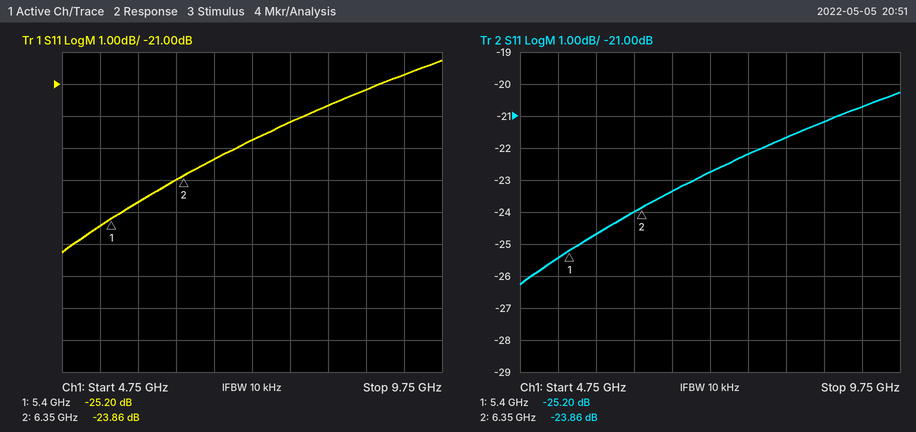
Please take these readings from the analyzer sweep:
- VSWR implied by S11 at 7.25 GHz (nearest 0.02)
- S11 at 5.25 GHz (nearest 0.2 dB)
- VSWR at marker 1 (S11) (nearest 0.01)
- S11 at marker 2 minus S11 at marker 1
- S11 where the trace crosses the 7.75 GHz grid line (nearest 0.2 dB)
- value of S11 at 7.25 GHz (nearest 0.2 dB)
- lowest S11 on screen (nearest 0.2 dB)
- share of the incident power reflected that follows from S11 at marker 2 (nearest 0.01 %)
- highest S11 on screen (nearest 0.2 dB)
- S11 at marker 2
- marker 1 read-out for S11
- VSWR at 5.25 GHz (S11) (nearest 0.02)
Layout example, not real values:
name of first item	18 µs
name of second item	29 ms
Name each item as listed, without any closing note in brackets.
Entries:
VSWR implied by S11 at 7.25 GHz	1.16
S11 at 5.25 GHz	-25.4 dB
VSWR at marker 1 (S11)	1.12
S11 at marker 2 minus S11 at marker 1	1.34 dB
S11 where the trace crosses the 7.75 GHz grid line	-22.2 dB
value of S11 at 7.25 GHz	-22.8 dB
lowest S11 on screen	-26.2 dB
share of the incident power reflected that follows from S11 at marker 2	0.41 %
highest S11 on screen	-20.2 dB
S11 at marker 2	-23.86 dB
marker 1 read-out for S11	-25.20 dB
VSWR at 5.25 GHz (S11)	1.12
